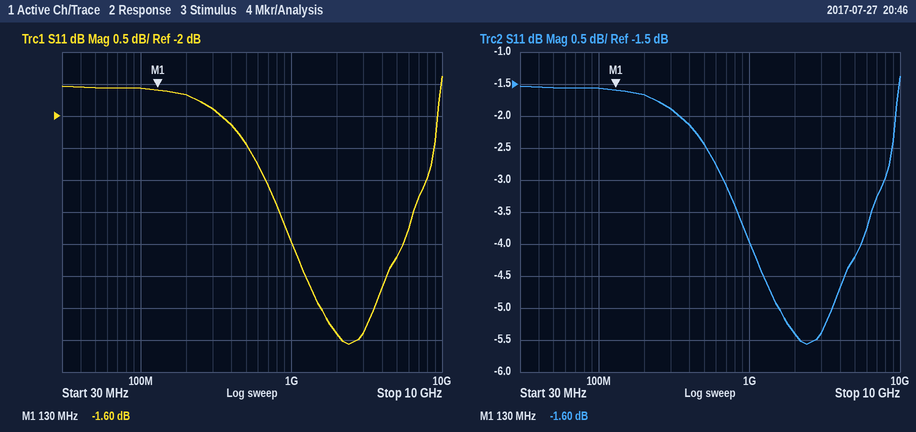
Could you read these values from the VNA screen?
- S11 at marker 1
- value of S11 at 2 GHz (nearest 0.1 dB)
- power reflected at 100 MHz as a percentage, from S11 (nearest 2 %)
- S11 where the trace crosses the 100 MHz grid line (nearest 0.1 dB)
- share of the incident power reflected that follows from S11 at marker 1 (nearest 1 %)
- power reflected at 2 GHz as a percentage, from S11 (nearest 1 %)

-1.60 dB
-5.4 dB
70 %
-1.6 dB
69 %
29 %
